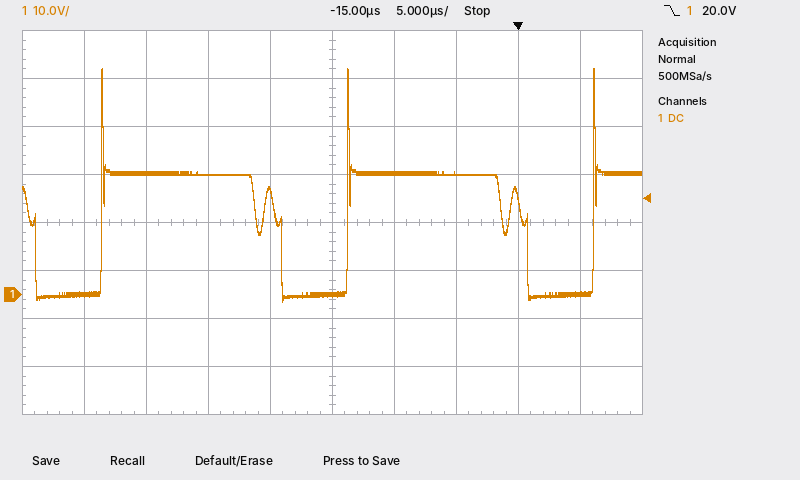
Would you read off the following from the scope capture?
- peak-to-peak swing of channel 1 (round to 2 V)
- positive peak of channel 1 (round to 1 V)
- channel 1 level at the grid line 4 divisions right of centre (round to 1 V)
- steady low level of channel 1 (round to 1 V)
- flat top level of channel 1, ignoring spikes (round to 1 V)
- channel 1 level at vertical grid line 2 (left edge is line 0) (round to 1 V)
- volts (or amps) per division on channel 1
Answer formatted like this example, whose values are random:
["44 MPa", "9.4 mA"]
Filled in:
["48 V", "47 V", "0 V", "0 V", "25 V", "25 V", "10 V"]
